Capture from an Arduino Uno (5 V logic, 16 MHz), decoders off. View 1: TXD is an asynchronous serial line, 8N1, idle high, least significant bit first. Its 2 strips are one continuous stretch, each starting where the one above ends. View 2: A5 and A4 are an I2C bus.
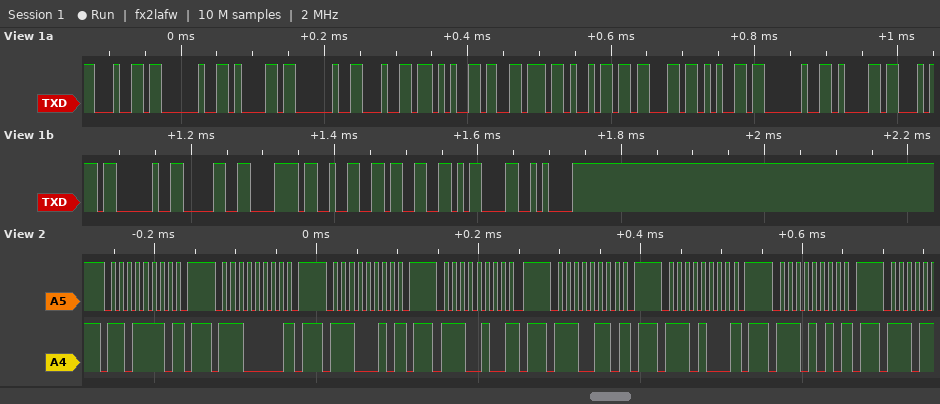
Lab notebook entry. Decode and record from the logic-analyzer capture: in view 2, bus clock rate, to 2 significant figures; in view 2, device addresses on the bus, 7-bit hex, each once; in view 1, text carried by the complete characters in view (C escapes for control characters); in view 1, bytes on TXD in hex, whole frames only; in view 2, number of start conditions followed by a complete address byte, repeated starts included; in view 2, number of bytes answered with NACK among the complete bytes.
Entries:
100 kHz
0x6F 0x70 0x71 0x72 0x73 0x74 0x75
"d a device at 0x23\r\n"
64 20 61 20 64 65 76 69 63 65 20 61 74 20 30 78 32 33 0D 0A
7
7
